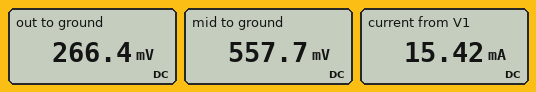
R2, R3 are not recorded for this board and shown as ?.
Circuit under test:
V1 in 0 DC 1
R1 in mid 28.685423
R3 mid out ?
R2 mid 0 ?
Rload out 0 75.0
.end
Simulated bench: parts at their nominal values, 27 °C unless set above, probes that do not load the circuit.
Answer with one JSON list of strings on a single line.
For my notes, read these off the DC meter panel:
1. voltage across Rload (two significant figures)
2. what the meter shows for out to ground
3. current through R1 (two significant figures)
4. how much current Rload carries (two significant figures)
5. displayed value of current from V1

["270 mV", "266.4 mV", "15 mA", "3.6 mA", "15.42 mA"]
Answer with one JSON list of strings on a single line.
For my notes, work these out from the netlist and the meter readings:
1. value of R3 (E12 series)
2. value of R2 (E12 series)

["82 Ω", "47 Ω"]
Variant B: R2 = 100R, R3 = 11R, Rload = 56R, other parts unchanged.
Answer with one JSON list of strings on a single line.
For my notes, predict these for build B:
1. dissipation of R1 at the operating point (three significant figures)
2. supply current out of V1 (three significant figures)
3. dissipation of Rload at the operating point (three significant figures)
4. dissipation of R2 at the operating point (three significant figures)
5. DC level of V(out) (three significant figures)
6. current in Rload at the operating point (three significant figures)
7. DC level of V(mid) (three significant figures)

["6.06 mW", "14.5 mA", "4.24 mW", "3.40 mW", "487 mV", "8.70 mA", "583 mV"]
